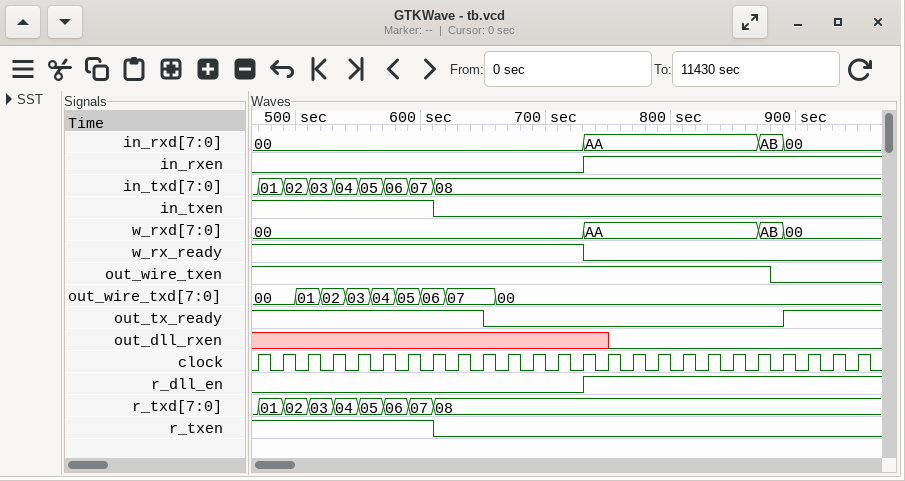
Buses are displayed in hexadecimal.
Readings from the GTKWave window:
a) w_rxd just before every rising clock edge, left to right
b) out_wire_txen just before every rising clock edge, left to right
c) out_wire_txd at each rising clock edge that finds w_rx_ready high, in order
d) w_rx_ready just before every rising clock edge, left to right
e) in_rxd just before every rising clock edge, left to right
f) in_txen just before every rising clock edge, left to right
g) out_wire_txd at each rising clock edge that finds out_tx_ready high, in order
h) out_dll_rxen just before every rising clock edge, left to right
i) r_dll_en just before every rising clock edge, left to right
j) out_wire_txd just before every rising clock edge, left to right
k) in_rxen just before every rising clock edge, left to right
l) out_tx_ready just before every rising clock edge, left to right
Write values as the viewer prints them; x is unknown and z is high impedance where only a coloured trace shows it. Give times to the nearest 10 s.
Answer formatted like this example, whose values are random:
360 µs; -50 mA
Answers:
00, 00, 00, 00, 00, 00, 00, 00, 00, 00, 00, 00, 00, 00, AA, AA, AA, AA, AA, AA, AA, AB, 00, 00, 00; 1 1 1 1 1 1 1 1 1 1 1 1 1 1 1 1 1 1 1 1 1 0 0 0 0; 00, 00, 01, 02, 03, 04, 05, 06, 07, 07, 00, 00, 00, 00; 1 1 1 1 1 1 1 1 1 1 1 1 1 1 0 0 0 0 0 0 0 0 0 0 0; 00, 00, 00, 00, 00, 00, 00, 00, 00, 00, 00, 00, 00, 00, AA, AA, AA, AA, AA, AA, AA, AB, 00, 00, 00; 1 1 1 1 1 1 1 1 0 0 0 0 0 0 0 0 0 0 0 0 0 0 0 0 0; 00, 00, 01, 02, 03, 04, 05, 06, 07, 07, 00, 00, 00; x x x x x x x x x x x x x x x 0 0 0 0 0 0 0 0 0 0; 0 0 0 0 0 0 0 0 0 0 0 0 0 0 1 1 1 1 1 1 1 1 1 1 1; 00, 00, 01, 02, 03, 04, 05, 06, 07, 07, 00, 00, 00, 00, 00, 00, 00, 00, 00, 00, 00, 00, 00, 00, 00; 0 0 0 0 0 0 0 0 0 0 0 0 0 0 1 1 1 1 1 1 1 1 1 1 1; 1 1 1 1 1 1 1 1 1 1 0 0 0 0 0 0 0 0 0 0 0 0 1 1 1
